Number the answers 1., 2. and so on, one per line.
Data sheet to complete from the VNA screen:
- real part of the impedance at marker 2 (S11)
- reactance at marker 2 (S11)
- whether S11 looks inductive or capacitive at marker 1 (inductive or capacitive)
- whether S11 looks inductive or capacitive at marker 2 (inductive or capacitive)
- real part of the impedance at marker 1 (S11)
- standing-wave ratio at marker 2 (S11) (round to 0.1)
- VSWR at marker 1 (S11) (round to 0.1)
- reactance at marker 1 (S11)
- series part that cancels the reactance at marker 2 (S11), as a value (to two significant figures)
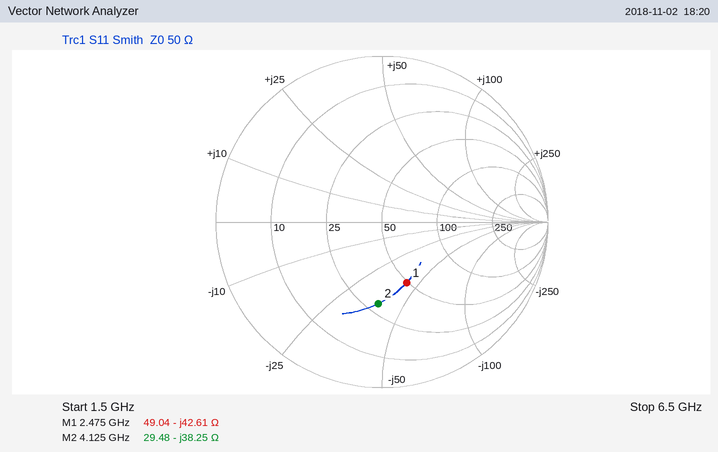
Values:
1. 29.48 Ω
2. -38.25 Ω
3. capacitive
4. capacitive
5. 49.04 Ω
6. 2.9
7. 2.3
8. -42.61 Ω
9. 1.5 nH
